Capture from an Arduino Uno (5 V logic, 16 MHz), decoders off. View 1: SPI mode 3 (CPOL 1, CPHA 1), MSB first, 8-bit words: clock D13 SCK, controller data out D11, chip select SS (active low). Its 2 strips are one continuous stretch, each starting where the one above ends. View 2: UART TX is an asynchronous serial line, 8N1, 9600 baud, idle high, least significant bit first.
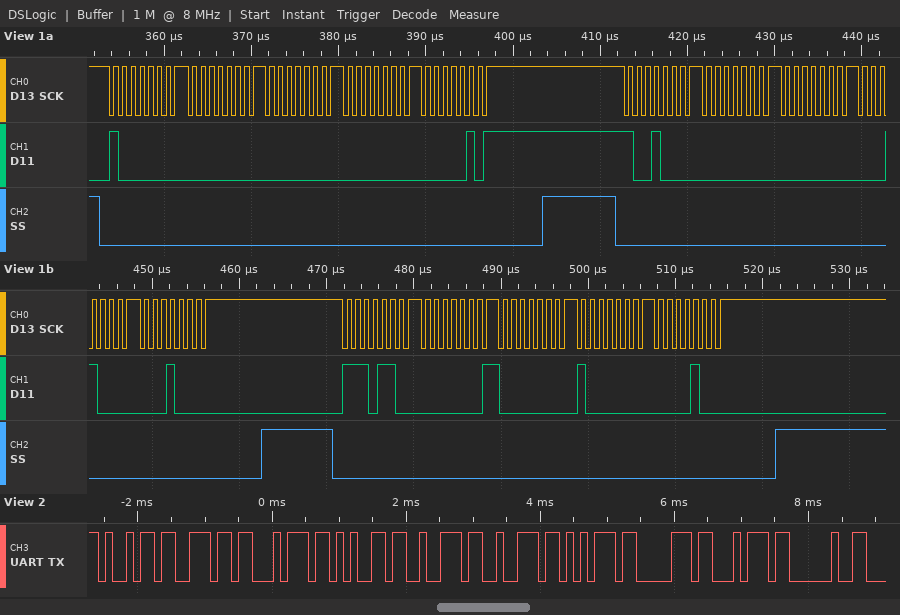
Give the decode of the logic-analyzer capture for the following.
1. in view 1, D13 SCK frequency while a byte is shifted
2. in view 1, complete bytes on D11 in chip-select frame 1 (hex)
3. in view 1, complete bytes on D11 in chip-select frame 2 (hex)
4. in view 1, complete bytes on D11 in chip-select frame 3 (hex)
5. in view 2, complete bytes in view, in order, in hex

1 MHz
80 00 00 00 05
90 00 00 10 10
EC 01 00 80 08
69 6E 74 65 72 72 75 70 74 20
